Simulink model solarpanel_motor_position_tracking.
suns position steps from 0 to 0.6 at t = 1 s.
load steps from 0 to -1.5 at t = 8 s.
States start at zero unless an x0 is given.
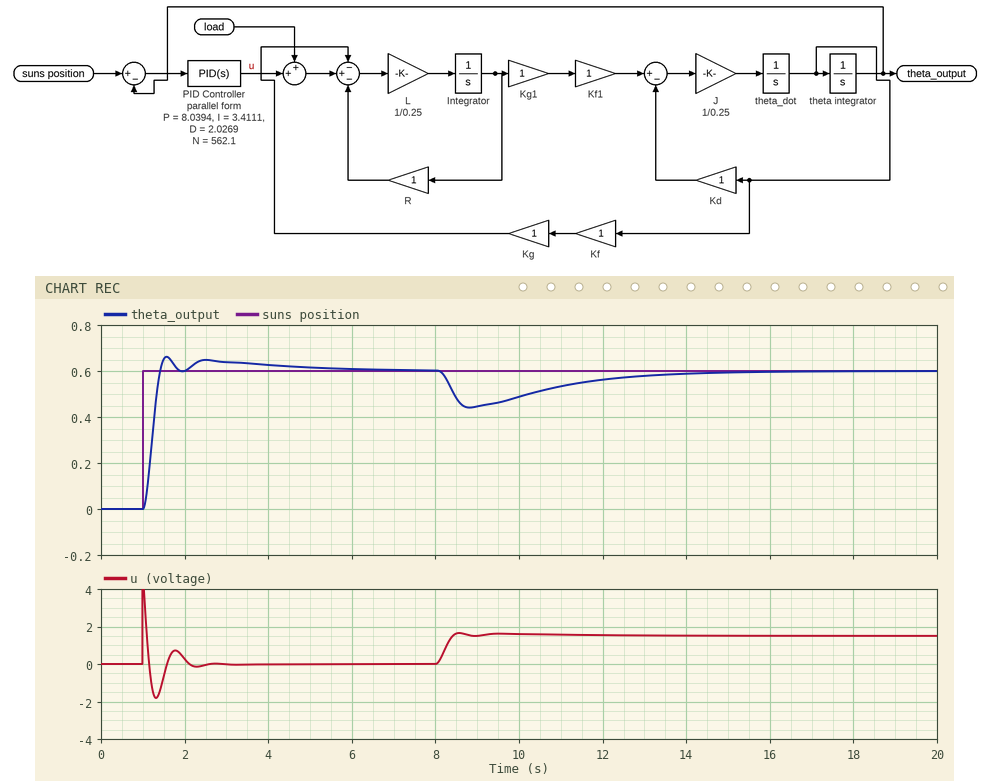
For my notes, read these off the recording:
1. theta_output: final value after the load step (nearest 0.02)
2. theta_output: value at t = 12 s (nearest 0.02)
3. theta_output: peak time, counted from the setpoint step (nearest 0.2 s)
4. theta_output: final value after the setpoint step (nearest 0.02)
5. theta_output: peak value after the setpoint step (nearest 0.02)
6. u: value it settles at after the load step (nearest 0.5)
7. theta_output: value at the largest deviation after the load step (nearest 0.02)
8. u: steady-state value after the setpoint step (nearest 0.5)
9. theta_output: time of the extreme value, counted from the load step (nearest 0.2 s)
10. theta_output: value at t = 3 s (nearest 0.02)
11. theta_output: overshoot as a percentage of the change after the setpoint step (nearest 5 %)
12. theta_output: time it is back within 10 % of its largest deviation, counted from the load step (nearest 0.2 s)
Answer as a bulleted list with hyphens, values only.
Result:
- 0.60
- 0.56
- 0.6 s
- 0.60
- 0.66
- 1.5
- 0.44
- 0.0
- 0.8 s
- 0.64
- 10 %
- 5.4 s
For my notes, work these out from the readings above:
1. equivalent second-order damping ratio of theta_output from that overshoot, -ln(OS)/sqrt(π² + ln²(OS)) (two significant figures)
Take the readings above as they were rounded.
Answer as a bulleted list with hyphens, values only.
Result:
- 0.59
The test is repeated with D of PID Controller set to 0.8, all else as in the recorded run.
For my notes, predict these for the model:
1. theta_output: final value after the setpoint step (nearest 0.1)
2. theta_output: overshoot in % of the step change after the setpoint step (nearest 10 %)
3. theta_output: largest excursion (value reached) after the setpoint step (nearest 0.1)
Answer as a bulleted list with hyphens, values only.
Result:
- 0.6
- 30 %
- 0.8
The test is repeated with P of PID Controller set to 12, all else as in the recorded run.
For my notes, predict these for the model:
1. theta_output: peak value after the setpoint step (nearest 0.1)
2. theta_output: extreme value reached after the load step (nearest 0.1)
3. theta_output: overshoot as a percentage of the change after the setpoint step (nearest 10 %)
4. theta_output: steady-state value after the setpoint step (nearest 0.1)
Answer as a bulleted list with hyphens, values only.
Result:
- 0.8
- 0.5
- 30 %
- 0.6
